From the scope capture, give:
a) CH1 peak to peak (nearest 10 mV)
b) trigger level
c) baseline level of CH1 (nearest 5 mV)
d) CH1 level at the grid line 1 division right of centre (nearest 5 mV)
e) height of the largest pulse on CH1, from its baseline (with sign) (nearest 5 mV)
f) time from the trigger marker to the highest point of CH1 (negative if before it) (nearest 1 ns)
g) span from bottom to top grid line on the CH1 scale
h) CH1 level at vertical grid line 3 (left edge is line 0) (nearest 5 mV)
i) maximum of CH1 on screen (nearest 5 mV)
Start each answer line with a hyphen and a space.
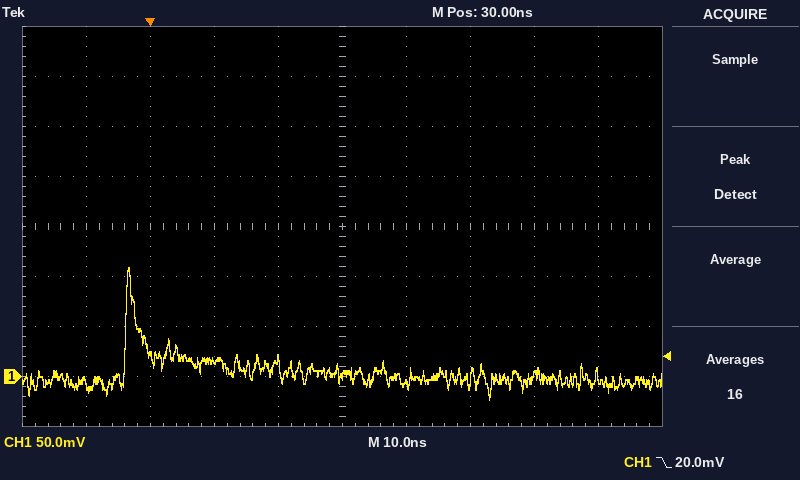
- 130 mV
- 20.0 mV
- 0 mV
- -10 mV
- +110 mV
- -3 ns
- 400 mV
- 15 mV
- 110 mV
